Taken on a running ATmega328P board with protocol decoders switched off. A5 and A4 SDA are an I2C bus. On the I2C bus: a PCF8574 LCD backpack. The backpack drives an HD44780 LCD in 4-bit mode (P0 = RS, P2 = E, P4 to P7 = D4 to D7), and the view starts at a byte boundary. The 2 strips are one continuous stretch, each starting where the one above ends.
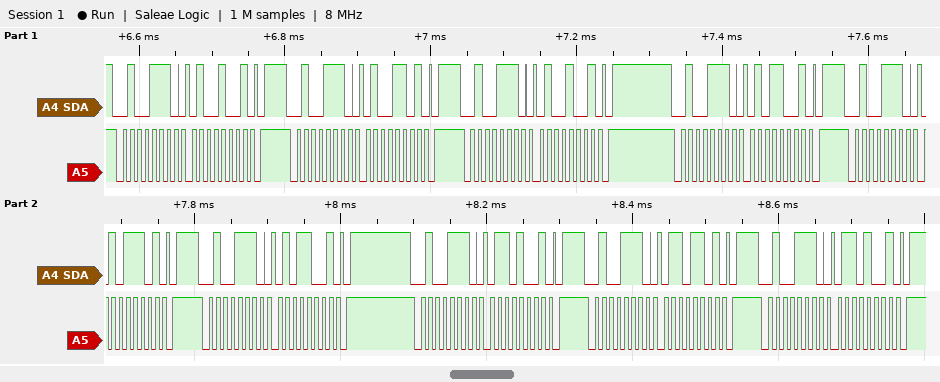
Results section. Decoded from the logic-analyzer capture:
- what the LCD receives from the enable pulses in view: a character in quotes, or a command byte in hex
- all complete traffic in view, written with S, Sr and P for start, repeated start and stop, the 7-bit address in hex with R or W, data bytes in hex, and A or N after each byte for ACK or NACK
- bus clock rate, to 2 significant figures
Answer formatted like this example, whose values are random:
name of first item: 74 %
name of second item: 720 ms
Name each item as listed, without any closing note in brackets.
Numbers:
what the LCD receives from the enable pulses in view: a character in quotes, or a command byte in hex: 'E'
all complete traffic in view, written with S, Sr and P for start, repeated start and stop, the 7-bit address in hex with R or W, data bytes in hex, and A or N after each byte for ACK or NACK: S 27W A 49 A P S 27W A 4D A P S 27W A 49 A P S 27W A 59 A P S 27W A 5D A P S 27W A 59 A P S 27W A 69 A P S 27W A 6D A P S 27W A 69 A P
bus clock rate, to 2 significant figures: 100 kHz
